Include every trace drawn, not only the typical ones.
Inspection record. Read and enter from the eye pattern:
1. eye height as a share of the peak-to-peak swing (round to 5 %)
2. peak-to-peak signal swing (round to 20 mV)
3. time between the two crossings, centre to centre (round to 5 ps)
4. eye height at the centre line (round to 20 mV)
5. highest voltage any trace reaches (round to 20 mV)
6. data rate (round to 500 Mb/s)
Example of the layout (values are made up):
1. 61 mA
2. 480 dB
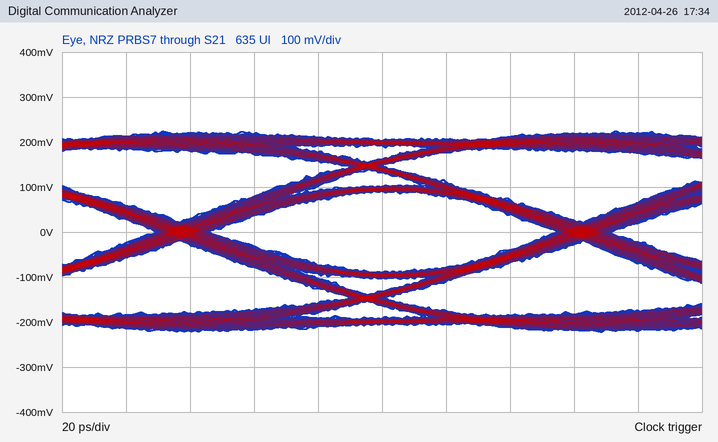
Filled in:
1. 40 %
2. 440 mV
3. 125 ps
4. 180 mV
5. 220 mV
6. 8.0 Gb/s
